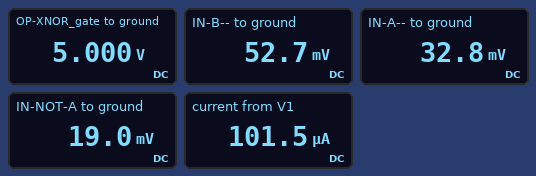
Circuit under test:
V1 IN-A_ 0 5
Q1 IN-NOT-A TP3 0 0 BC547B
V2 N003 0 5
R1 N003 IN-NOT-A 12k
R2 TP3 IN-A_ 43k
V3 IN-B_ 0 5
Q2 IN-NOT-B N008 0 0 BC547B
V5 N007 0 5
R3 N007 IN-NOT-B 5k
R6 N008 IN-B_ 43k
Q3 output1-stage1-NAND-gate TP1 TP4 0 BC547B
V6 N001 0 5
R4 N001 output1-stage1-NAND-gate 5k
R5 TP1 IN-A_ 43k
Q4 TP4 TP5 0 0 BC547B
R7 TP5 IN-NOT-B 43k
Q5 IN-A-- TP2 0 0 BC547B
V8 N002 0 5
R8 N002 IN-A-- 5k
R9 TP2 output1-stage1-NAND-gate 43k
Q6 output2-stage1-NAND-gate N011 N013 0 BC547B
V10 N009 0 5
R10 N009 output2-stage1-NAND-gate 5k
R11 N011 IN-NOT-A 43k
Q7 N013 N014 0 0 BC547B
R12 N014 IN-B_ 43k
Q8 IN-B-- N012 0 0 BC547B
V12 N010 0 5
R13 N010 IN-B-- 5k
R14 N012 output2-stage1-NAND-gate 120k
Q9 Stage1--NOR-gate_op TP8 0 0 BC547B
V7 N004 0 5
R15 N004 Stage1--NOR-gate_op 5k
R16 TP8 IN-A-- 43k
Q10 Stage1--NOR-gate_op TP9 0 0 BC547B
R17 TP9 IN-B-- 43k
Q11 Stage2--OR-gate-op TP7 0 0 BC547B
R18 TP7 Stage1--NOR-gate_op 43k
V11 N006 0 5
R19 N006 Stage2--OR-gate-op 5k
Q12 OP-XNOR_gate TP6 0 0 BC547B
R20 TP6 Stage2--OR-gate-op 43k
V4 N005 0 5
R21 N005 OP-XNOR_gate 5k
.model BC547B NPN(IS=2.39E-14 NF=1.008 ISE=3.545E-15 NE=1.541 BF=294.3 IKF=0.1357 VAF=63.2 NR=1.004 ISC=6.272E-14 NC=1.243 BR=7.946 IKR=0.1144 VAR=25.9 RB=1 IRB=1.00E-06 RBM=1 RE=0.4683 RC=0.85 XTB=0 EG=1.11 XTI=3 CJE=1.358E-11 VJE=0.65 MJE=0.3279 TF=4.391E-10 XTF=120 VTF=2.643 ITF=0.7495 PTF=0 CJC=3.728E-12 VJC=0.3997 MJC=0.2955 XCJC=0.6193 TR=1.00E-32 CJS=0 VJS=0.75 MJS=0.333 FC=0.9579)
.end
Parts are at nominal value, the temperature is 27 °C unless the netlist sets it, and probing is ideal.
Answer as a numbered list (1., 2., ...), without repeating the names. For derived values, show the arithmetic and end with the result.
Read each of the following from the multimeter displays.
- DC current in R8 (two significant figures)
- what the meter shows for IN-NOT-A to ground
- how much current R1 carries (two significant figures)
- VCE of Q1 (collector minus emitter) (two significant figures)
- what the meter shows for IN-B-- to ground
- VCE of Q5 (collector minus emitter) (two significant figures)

1. (5 V - 32.8 mV) / 5 kΩ = 990 µA
2. 19.0 mV
3. (5 V - 19 mV) / 12 kΩ = 420 µA
4. 19 mV = 19 mV
5. 52.7 mV
6. 32.8 mV = 33 mV
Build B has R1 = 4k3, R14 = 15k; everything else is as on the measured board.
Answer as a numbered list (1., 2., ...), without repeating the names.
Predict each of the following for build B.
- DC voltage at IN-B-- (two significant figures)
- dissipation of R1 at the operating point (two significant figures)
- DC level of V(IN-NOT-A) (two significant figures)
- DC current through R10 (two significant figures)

1. 21 mV
2. 5.7 mW
3. 34 mV
4. 220 µA
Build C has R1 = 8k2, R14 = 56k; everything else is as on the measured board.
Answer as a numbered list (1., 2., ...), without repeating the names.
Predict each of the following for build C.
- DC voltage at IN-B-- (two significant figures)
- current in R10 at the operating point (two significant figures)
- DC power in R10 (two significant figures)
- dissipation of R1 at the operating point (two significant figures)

1. 37 mV
2. 71 µA
3. 25 µW
4. 3.0 mW
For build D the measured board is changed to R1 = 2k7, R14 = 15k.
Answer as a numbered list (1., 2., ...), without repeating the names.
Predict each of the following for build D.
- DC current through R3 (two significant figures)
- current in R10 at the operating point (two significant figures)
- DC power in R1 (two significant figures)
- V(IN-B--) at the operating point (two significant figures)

1. 990 µA
2. 220 µA
3. 9.1 mW
4. 21 mV
